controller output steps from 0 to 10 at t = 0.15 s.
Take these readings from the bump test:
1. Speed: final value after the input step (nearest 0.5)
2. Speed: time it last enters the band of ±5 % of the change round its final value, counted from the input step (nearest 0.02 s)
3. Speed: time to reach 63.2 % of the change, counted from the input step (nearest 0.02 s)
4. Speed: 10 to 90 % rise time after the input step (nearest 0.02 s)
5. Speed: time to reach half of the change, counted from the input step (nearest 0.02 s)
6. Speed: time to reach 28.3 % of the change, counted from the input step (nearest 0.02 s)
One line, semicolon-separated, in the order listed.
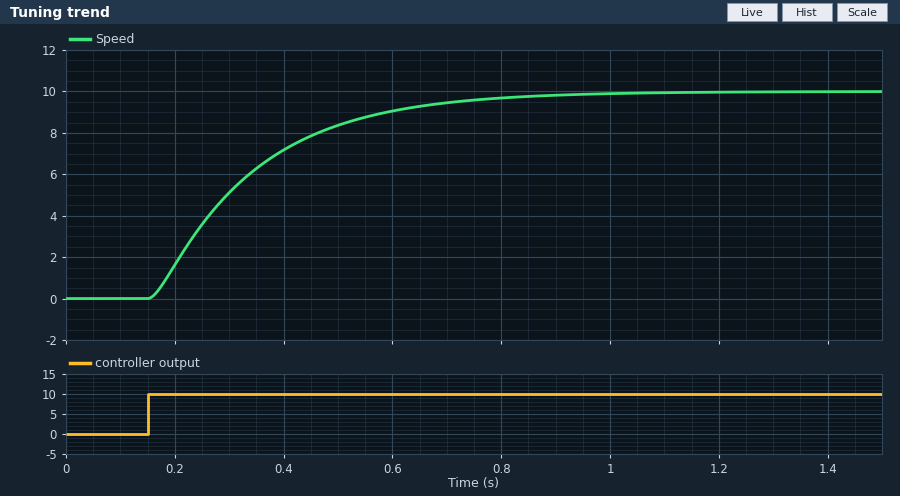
10.0; 0.56 s; 0.20 s; 0.40 s; 0.14 s; 0.08 s
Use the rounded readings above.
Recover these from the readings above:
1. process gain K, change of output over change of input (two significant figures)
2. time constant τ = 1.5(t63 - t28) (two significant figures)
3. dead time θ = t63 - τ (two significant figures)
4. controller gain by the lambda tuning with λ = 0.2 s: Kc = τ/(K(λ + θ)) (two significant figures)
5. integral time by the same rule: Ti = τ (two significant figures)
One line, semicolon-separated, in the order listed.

1.0; 0.18 s; 0.020 s; 0.82; 0.18 s
